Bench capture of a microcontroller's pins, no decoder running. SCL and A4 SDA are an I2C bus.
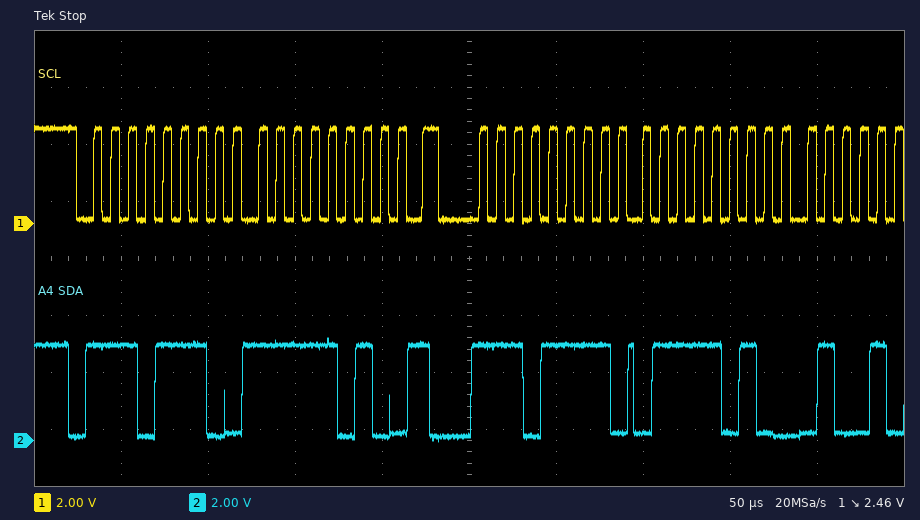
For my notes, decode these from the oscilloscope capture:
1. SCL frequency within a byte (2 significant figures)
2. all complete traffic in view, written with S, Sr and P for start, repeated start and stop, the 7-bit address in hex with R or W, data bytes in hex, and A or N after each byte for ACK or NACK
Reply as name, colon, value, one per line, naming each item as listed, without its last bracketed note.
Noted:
SCL frequency within a byte: 100 kHz
all complete traffic in view, written with S, Sr and P for start, repeated start and stop, the 7-bit address in hex with R or W, data bytes in hex, and A or N after each byte for ACK or NACK: S 77W A FA A Sr 77R A 7A A
